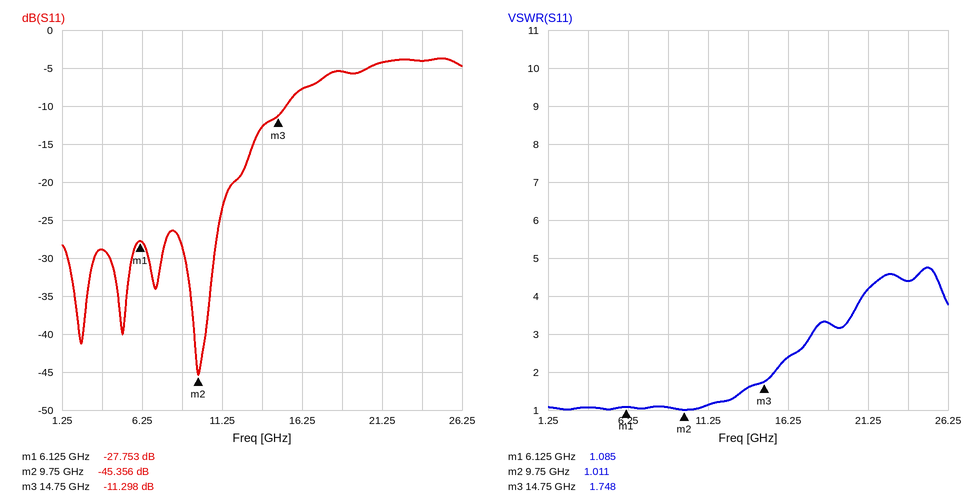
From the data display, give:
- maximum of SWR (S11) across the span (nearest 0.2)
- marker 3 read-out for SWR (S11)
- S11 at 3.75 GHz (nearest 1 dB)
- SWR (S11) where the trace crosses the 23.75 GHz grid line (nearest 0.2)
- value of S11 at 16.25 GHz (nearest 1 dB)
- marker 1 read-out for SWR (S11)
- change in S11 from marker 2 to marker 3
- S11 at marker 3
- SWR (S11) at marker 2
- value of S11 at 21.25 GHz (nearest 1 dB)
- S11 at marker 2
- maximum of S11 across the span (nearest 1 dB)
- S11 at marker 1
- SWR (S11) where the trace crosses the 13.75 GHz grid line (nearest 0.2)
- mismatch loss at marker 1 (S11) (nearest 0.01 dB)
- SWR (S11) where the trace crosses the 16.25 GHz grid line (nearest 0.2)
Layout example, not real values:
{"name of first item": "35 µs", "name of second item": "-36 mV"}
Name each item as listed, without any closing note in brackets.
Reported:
{"maximum of SWR (S11) across the span": "4.8", "marker 3 read-out for SWR": "1.748", "S11 at 3.75 GHz": "-29 dB", "SWR (S11) where the trace crosses the 23.75 GHz grid line": "4.4", "value of S11 at 16.25 GHz": "-8 dB", "marker 1 read-out for SWR": "1.085", "change in S11 from marker 2 to marker 3": "34.058 dB", "S11 at marker 3": "-11.298 dB", "SWR (S11) at marker 2": "1.011", "value of S11 at 21.25 GHz": "-4 dB", "S11 at marker 2": "-45.356 dB", "maximum of S11 across the span": "-4 dB", "S11 at marker 1": "-27.753 dB", "SWR (S11) where the trace crosses the 13.75 GHz grid line": "1.6", "mismatch loss at marker 1 (S11)": "0.01 dB", "SWR (S11) where the trace crosses the 16.25 GHz grid line": "2.4"}
